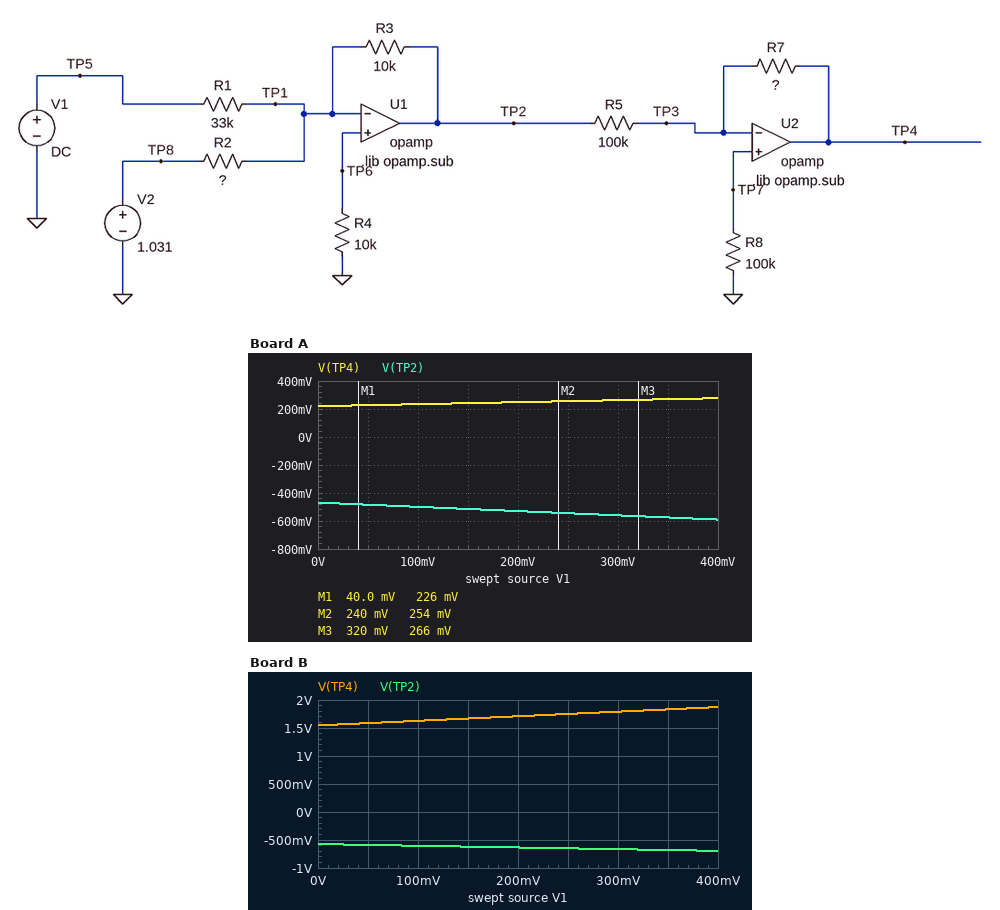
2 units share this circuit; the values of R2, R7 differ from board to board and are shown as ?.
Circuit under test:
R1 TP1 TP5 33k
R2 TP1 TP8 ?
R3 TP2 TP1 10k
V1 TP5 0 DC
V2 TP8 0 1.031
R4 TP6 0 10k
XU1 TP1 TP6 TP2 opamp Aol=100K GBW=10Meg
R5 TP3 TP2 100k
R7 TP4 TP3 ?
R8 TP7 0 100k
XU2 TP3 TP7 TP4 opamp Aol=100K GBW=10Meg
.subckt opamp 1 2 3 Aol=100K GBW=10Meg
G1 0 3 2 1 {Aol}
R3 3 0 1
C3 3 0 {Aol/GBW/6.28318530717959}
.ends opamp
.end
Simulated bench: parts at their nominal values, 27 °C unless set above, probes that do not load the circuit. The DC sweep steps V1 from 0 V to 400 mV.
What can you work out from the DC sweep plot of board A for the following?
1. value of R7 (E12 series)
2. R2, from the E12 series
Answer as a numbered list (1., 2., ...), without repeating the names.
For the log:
1. 47 kΩ
2. 22 kΩ
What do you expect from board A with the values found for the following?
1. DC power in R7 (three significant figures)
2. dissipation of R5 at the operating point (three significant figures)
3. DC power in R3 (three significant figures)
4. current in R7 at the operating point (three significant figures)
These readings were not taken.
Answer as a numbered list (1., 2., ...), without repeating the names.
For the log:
1. 1.03 µW
2. 2.20 µW
3. 22.0 µW
4. 4.69 µA
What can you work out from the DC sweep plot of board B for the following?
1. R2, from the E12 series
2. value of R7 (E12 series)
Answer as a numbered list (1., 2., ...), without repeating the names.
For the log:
1. 18 kΩ
2. 270 kΩ
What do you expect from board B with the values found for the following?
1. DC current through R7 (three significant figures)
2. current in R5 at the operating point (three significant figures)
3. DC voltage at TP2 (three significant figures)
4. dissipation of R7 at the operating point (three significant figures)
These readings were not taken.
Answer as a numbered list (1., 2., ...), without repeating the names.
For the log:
1. 5.73 µA
2. 5.73 µA
3. -573 mV
4. 8.86 µW
